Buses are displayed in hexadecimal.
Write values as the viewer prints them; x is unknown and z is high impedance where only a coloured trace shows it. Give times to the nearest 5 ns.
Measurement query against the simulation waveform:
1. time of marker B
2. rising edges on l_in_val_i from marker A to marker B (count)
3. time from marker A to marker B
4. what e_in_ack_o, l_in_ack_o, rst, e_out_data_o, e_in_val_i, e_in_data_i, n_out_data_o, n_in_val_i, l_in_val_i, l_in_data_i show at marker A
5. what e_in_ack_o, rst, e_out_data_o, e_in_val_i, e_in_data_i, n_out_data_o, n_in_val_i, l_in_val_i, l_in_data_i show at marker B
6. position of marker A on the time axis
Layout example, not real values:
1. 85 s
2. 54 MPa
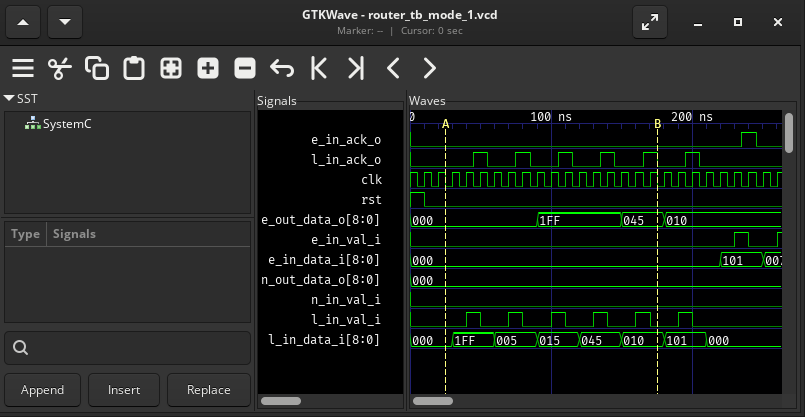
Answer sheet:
1. 175 ns
2. 5
3. 150 ns
4. e_in_ack_o=0, l_in_ack_o=0, rst=0, e_out_data_o=000, e_in_val_i=0, e_in_data_i=000, n_out_data_o=000, n_in_val_i=0, l_in_val_i=0, l_in_data_i=000
5. e_in_ack_o=0, rst=0, e_out_data_o=045, e_in_val_i=0, e_in_data_i=000, n_out_data_o=000, n_in_val_i=0, l_in_val_i=0, l_in_data_i=010
6. 25 ns
